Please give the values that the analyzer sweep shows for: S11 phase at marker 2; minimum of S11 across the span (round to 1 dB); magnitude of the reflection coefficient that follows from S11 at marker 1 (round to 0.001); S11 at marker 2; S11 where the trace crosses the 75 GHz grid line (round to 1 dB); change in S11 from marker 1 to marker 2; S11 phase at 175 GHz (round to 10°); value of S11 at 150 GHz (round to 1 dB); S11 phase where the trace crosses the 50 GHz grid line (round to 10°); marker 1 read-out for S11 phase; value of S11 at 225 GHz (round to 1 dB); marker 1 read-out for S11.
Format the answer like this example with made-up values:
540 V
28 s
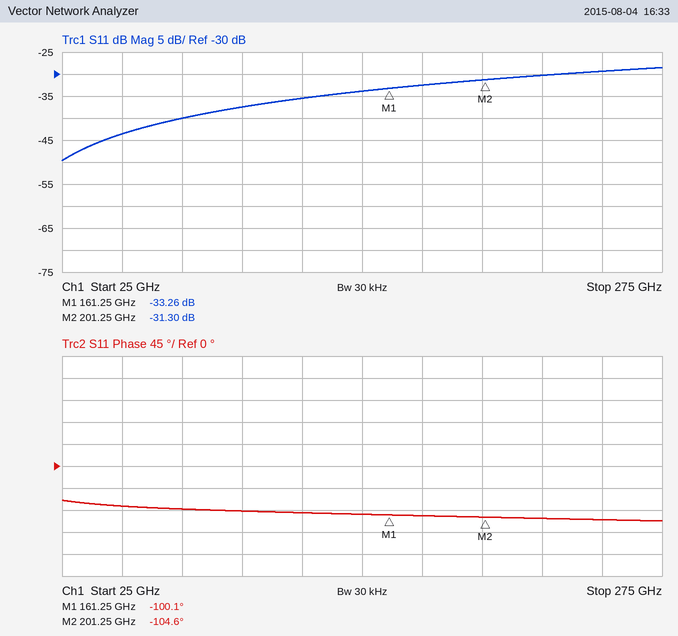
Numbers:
-104.6°
-50 dB
0.022
-31.30 dB
-40 dB
1.96 dB
-100°
-34 dB
-80°
-100.1°
-30 dB
-33.26 dB
